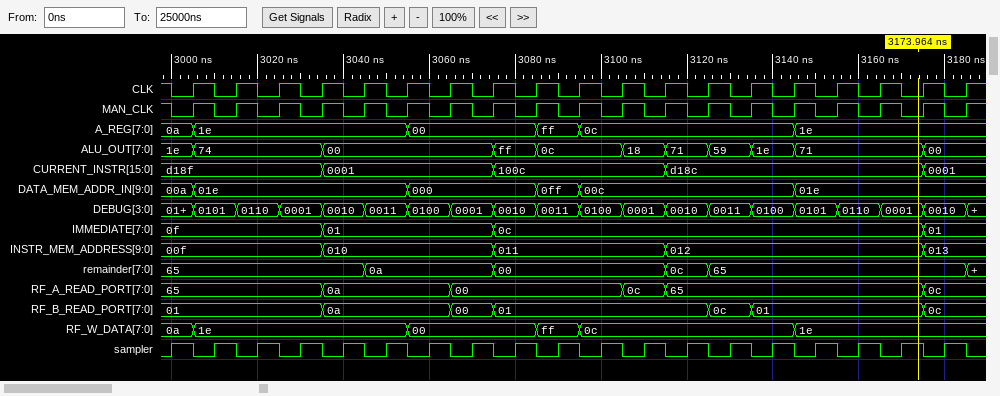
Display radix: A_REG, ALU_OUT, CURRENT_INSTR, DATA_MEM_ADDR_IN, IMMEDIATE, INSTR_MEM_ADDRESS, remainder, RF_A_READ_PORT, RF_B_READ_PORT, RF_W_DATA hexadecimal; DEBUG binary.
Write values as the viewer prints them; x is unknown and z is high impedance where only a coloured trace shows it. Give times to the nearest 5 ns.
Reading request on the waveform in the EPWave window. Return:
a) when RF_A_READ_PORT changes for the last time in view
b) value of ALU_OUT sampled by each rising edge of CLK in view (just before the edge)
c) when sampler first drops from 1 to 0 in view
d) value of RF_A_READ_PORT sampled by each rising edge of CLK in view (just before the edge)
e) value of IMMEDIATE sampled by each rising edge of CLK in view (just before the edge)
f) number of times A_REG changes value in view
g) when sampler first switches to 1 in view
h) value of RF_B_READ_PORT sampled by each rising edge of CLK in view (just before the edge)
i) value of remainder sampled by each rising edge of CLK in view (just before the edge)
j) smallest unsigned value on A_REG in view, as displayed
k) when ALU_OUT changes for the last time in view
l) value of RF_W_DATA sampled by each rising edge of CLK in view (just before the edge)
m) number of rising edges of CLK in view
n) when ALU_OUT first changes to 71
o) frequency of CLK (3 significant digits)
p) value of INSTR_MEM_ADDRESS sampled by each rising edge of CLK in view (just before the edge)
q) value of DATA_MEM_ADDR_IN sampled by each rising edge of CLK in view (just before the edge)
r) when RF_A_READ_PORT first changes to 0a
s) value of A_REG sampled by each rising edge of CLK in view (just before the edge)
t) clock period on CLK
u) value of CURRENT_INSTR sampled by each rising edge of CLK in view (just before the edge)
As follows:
3175 ns
1e, 74, 74, 74, 00, 00, 00, 00, ff, 0c, 0c, 18, 71, 59, 1e, 71, 71, 71, 00
3005 ns
65, 65, 65, 65, 0a, 0a, 0a, 00, 00, 00, 00, 0c, 65, 65, 65, 65, 65, 65, 0c
0f, 0f, 0f, 0f, 01, 01, 01, 01, 0c, 0c, 0c, 0c, 0c, 0c, 0c, 0c, 0c, 0c, 01
5
3000 ns
01, 01, 01, 01, 0a, 0a, 0a, 00, 01, 01, 01, 01, 01, 0c, 01, 01, 01, 01, 0c
65, 65, 65, 65, 65, 0a, 0a, 0a, 00, 00, 00, 00, 0c, 65, 65, 65, 65, 65, 65
00
3175 ns
0a, 1e, 1e, 1e, 1e, 1e, 00, 00, 00, ff, 0c, 0c, 0c, 0c, 0c, 1e, 1e, 1e, 1e
19
3115 ns
100 MHz
00f, 00f, 00f, 00f, 010, 010, 010, 010, 011, 011, 011, 011, 012, 012, 012, 012, 012, 012, 013
00a, 01e, 01e, 01e, 01e, 01e, 000, 000, 000, 0ff, 00c, 00c, 00c, 00c, 00c, 01e, 01e, 01e, 01e
3035 ns
0a, 1e, 1e, 1e, 1e, 1e, 00, 00, 00, ff, 0c, 0c, 0c, 0c, 0c, 1e, 1e, 1e, 1e
10 ns
d18f, d18f, d18f, d18f, 0001, 0001, 0001, 0001, 100c, 100c, 100c, 100c, d18c, d18c, d18c, d18c, d18c, d18c, 0001
